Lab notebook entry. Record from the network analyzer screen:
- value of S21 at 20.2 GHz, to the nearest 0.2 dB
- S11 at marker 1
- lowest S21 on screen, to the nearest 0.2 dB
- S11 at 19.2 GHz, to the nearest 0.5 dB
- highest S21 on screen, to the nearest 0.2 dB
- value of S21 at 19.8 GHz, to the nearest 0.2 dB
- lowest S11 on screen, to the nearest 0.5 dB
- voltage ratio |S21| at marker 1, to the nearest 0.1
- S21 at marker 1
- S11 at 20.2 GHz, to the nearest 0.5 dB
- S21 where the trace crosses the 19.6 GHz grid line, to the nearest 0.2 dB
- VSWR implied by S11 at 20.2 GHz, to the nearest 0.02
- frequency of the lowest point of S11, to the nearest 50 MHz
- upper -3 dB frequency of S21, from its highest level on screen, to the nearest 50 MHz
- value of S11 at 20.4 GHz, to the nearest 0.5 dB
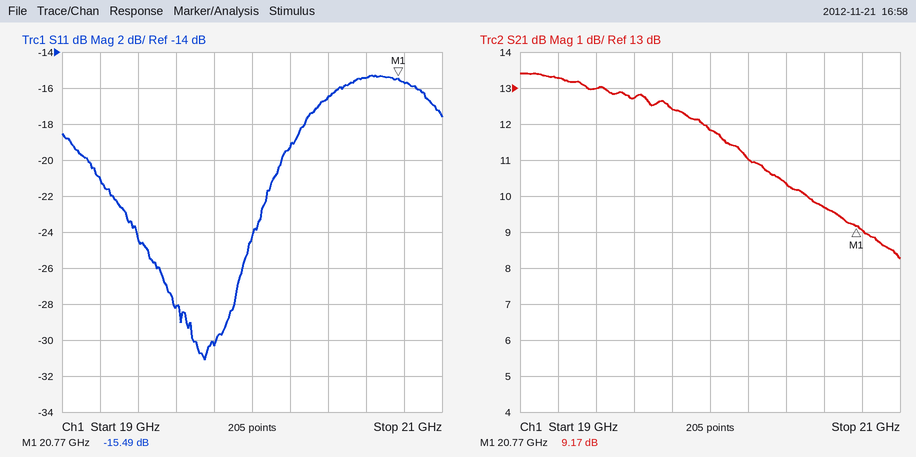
11.0 dB
-15.49 dB
8.2 dB
-21.0 dB
13.4 dB
12.4 dB
-31.0 dB
2.9
9.17 dB
-19.5 dB
12.8 dB
1.24
19.75 GHz
20.40 GHz
-16.5 dB
